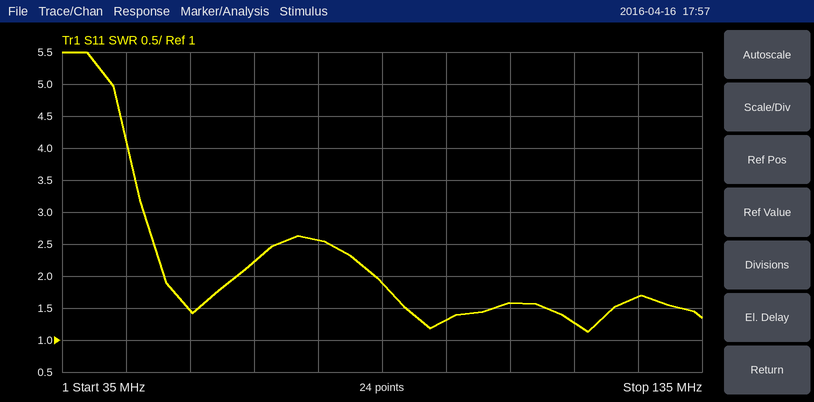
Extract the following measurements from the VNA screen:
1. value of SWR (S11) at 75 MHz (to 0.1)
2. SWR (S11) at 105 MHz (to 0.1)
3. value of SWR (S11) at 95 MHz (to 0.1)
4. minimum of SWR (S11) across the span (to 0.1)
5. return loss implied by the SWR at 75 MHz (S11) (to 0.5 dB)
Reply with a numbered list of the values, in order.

1. 2.6
2. 1.6
3. 1.3
4. 1.1
5. 7.0 dB
